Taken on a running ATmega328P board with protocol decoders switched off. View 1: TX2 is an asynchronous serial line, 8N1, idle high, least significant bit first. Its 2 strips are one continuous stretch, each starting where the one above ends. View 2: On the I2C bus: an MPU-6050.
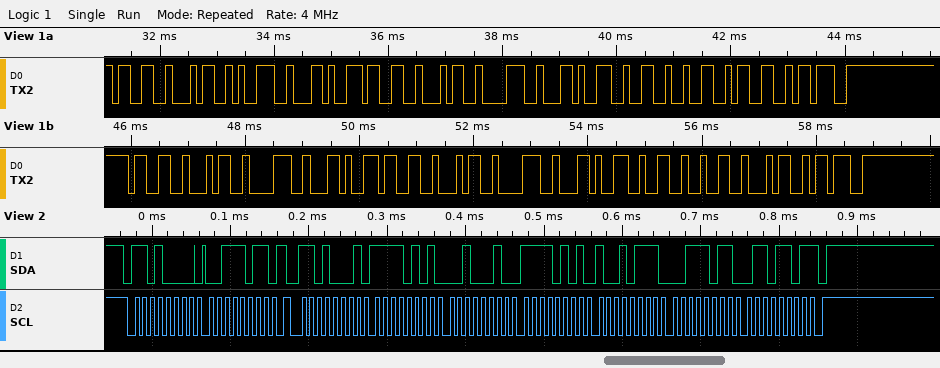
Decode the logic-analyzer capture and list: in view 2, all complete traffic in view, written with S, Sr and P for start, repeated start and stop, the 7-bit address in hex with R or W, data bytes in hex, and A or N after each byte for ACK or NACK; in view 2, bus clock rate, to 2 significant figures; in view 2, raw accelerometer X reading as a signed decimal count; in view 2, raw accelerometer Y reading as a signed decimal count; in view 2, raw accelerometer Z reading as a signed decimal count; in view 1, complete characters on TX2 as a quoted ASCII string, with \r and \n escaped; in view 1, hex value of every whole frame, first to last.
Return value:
S 68W A 3B A Sr 68R A F5 A 22 A F5 A 97 A 3B A 6D N P
100 kHz
-2782
-2665
15213
"349,348,223;348,348,224;"
33 34 39 2C 33 34 38 2C 32 32 33 3B 33 34 38 2C 33 34 38 2C 32 32 34 3B
